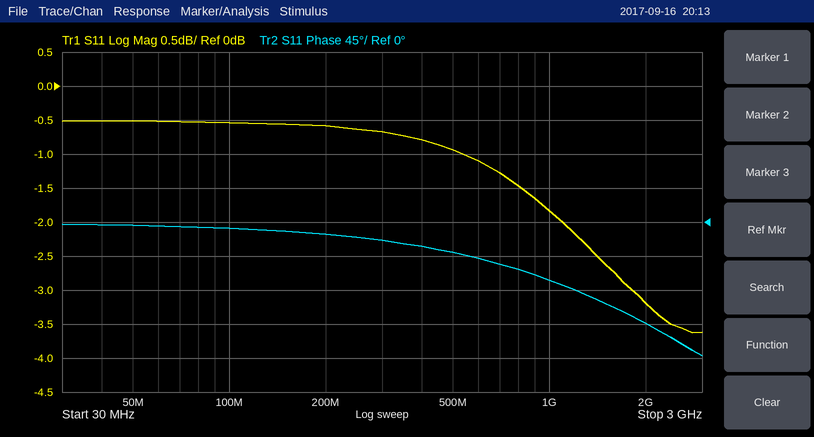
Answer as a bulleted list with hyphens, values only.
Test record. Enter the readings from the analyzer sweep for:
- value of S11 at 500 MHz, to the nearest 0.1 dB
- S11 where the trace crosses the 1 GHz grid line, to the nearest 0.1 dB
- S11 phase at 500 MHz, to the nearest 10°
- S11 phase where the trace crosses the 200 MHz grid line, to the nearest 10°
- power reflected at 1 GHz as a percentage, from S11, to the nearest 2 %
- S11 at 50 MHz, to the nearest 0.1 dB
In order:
- -0.9 dB
- -1.8 dB
- -40°
- -20°
- 66 %
- -0.5 dB
